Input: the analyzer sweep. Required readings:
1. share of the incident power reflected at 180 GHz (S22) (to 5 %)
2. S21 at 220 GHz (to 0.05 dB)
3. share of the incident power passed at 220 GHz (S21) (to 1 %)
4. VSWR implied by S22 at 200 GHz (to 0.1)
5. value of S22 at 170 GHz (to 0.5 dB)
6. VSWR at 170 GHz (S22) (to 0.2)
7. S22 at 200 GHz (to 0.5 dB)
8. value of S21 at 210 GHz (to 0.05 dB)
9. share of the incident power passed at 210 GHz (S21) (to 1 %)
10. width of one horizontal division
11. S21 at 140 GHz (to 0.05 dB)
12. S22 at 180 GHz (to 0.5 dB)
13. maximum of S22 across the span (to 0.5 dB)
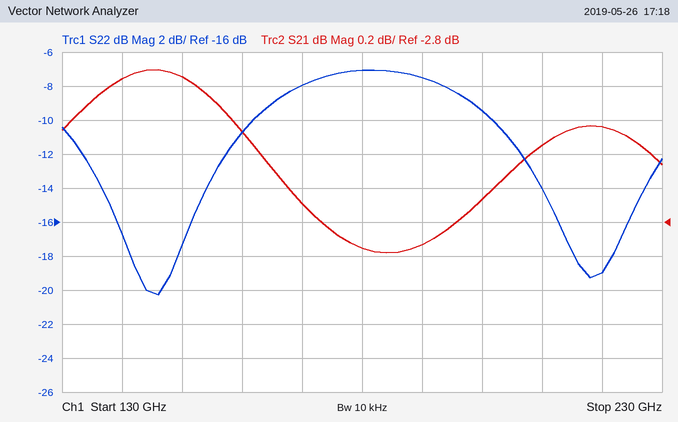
20 %
-2.25 dB
60 %
2.0
-8.0 dB
2.4
-9.5 dB
-2.35 dB
58 %
10 GHz
-1.95 dB
-7.0 dB
-7.0 dB
